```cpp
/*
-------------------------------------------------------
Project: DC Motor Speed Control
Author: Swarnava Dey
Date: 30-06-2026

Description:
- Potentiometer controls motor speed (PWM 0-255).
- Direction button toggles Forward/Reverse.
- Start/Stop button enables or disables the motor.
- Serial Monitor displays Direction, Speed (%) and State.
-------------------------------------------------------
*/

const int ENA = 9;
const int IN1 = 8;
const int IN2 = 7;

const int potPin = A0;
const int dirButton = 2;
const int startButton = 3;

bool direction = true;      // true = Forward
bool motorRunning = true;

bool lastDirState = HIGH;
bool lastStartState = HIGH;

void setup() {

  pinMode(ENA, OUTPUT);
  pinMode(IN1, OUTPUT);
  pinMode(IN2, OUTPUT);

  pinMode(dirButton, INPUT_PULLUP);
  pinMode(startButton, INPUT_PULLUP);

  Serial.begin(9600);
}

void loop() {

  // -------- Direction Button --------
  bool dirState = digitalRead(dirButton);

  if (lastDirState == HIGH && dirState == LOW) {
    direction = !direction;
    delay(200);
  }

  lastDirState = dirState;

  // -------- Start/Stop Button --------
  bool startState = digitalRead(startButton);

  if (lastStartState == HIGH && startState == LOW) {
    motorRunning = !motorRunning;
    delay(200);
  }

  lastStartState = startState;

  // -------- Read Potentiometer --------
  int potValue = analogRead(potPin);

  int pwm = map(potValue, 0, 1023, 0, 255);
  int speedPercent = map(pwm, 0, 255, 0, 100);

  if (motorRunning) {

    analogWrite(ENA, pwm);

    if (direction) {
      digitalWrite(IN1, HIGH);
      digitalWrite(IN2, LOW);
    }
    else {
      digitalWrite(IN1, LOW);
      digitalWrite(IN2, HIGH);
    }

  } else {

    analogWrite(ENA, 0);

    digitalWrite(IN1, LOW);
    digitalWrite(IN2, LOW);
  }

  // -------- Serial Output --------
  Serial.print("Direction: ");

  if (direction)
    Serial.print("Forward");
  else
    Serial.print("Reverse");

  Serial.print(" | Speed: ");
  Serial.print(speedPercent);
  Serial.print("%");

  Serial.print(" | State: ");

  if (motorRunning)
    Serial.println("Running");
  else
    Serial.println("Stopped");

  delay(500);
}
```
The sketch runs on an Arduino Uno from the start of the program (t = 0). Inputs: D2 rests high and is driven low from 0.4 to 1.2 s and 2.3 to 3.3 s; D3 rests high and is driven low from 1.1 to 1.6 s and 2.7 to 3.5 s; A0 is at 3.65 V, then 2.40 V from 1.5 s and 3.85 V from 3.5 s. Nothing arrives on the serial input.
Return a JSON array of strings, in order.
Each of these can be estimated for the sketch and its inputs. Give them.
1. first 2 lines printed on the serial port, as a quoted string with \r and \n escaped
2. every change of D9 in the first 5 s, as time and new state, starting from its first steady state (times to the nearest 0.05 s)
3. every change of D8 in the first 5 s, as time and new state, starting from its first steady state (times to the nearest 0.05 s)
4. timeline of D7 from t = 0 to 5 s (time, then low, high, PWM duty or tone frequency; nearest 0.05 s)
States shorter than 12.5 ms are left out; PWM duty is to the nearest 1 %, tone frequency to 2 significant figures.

["\"Direction: Forward | Speed: 72% | State: Running\\r\\nDirection: Reverse | Speed: 72% | State: Running\\r\\n\"", "0 s PWM 73 %; 1.4 s low; 3.3 s PWM 48 %; 3.8 s PWM 77 %", "0 s high; 0.7 s low; 3.3 s high", "0 s low; 0.7 s high; 1.4 s low"]
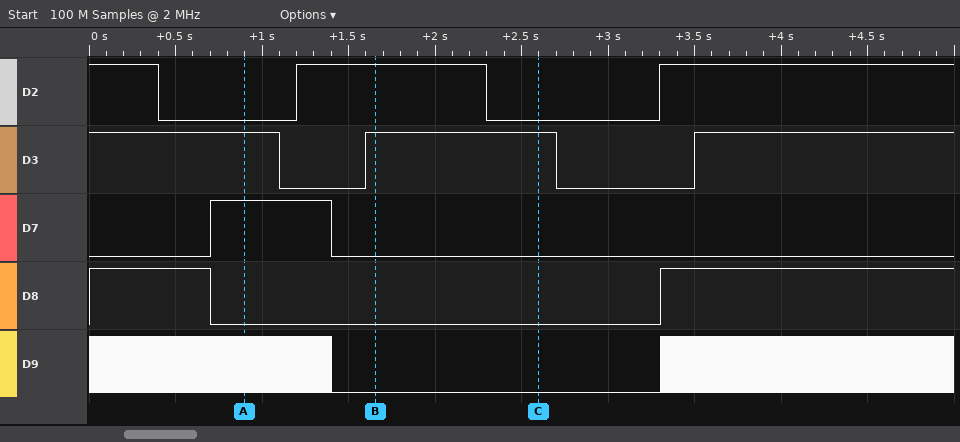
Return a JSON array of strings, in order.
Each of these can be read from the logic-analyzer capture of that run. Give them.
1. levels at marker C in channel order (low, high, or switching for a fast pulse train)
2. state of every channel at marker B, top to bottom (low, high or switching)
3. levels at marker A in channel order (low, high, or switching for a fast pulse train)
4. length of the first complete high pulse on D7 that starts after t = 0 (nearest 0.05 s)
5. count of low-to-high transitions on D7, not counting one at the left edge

["D2 low, D3 high, D7 low, D8 low, D9 low", "D2 high, D3 high, D7 low, D8 low, D9 low", "D2 low, D3 high, D7 high, D8 low, D9 switching", "0.70 s", "1"]
